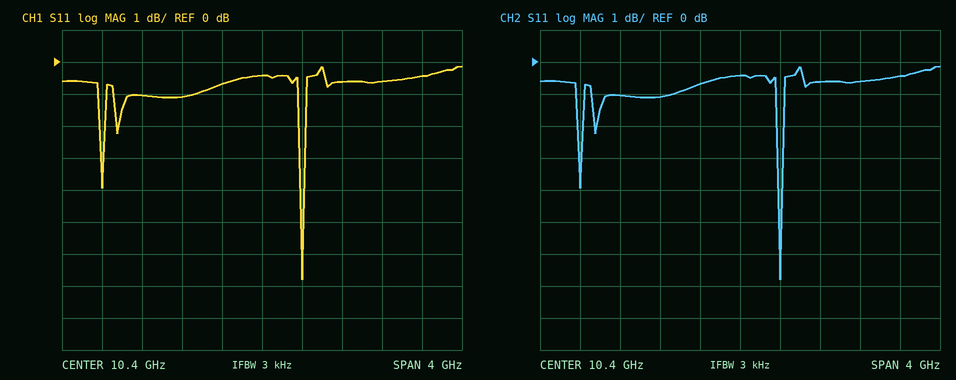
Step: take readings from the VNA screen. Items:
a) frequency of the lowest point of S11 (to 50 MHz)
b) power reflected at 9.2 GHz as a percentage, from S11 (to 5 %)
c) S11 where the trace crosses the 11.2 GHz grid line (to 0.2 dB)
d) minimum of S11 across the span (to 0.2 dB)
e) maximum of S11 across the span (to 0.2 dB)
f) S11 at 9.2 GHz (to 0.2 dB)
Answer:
10.80 GHz
80 %
-0.6 dB
-6.8 dB
-0.2 dB
-1.0 dB
